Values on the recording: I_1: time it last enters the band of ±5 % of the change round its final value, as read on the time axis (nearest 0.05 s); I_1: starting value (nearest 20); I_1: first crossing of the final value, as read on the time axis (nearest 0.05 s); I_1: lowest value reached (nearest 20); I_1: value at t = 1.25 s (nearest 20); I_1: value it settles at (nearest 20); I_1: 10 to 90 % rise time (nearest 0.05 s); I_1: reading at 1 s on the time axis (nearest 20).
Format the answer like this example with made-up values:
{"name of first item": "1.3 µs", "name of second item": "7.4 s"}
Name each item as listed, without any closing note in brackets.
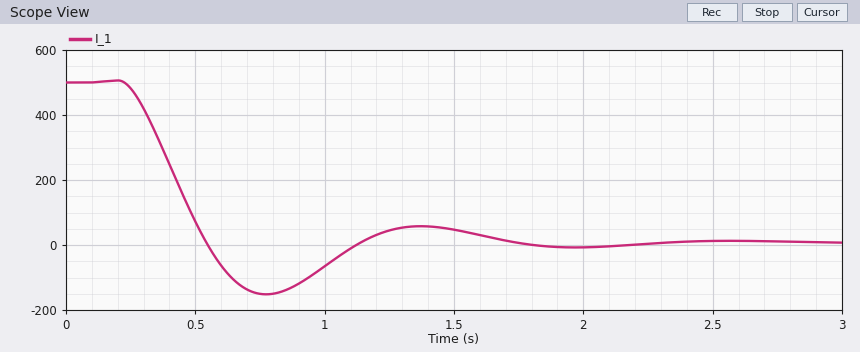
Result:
{"I_1: time it last enters the band of ±5 % of the change round its final value, as read on the time axis": "1.60 s", "I_1: starting value": "500", "I_1: first crossing of the final value, as read on the time axis": "0.55 s", "I_1: lowest value reached": "-160", "I_1: value at t = 1.25 s": "40", "I_1: value it settles at": "0", "I_1: 10 to 90 % rise time": "0.25 s", "I_1: reading at 1 s on the time axis": "-60"}
